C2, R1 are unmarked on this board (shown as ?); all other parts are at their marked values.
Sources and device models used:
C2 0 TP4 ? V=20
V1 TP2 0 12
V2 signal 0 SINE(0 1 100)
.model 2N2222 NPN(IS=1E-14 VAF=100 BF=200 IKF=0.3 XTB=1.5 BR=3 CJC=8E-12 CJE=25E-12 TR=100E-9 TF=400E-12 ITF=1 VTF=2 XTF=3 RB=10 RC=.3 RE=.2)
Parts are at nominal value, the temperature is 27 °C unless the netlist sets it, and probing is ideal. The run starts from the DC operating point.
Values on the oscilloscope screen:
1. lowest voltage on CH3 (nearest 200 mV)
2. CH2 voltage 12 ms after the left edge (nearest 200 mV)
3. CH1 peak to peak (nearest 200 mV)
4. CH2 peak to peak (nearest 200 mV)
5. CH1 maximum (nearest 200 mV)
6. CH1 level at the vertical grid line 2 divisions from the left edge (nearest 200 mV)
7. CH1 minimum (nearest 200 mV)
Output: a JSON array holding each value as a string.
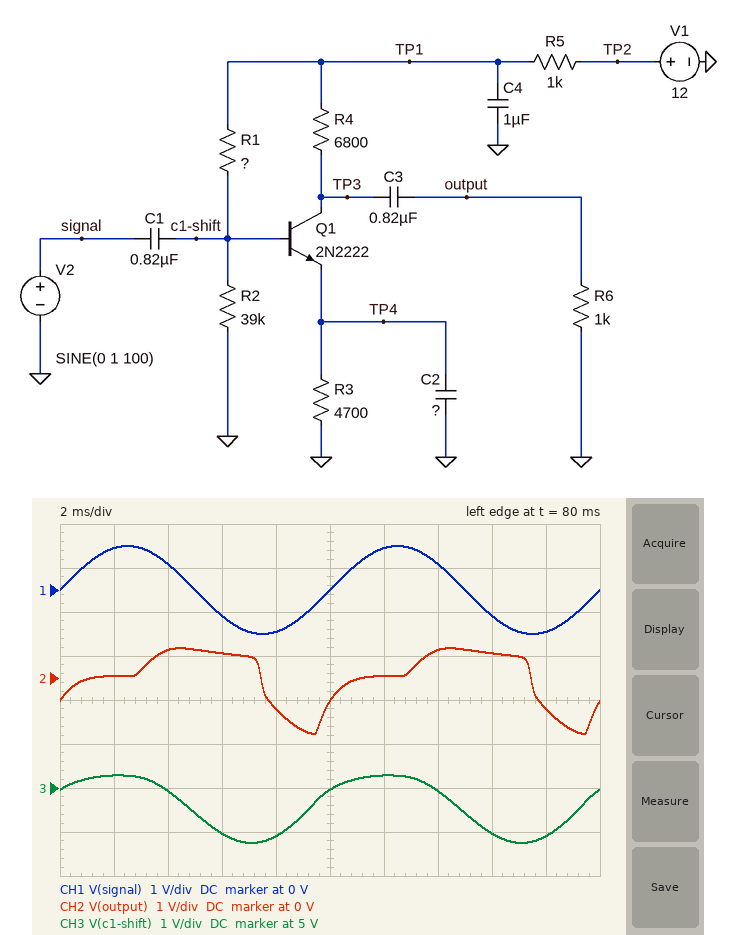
["3.8 V", "0 V", "2.0 V", "2.0 V", "1.0 V", "600 mV", "-1.0 V"]
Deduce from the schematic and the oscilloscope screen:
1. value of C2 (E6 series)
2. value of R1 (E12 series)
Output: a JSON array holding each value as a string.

["2.2 µF", "33 kΩ"]
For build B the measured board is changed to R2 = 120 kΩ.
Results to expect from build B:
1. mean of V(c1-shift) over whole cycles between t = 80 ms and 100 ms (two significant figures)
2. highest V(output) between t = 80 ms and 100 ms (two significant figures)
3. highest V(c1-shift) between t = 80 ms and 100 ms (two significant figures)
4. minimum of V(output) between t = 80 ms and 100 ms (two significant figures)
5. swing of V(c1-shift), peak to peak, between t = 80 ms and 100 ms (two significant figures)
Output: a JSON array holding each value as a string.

["5.1 V", "620 mV", "5.6 V", "-1.2 V", "1.2 V"]
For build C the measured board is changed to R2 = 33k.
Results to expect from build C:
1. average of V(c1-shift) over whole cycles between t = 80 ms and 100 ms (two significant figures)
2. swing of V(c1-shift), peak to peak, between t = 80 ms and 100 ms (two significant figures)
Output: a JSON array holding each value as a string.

["4.5 V", "1.6 V"]
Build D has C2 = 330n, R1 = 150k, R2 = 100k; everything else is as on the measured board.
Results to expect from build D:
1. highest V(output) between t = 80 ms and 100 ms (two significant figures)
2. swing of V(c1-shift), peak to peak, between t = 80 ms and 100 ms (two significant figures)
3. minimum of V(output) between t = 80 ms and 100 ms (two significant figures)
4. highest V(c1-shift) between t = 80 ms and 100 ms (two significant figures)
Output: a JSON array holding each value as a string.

["250 mV", "2.0 V", "-250 mV", "5.2 V"]
